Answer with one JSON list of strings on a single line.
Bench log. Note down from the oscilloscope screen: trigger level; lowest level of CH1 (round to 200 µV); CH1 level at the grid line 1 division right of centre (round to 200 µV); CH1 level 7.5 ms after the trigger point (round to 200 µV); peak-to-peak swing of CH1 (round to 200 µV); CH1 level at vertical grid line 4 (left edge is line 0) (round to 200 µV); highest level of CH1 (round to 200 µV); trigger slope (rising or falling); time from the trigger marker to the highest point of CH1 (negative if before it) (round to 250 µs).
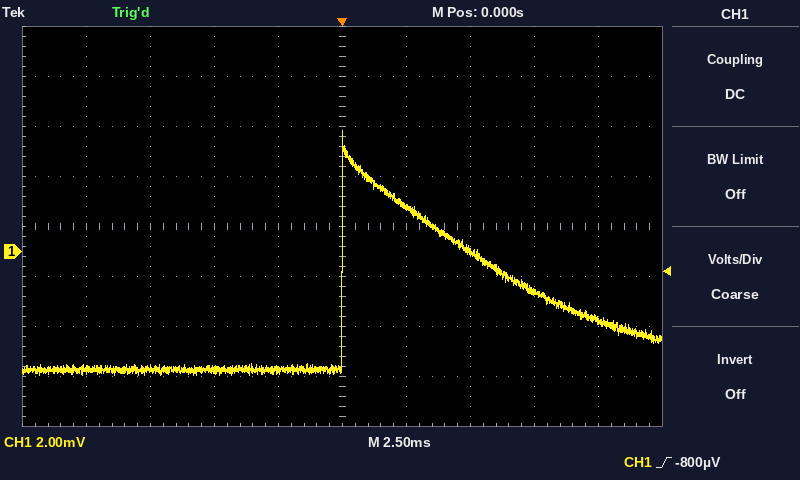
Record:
["-800 µV", "-5.0 mV", "1.8 mV", "-1.6 mV", "9.8 mV", "-4.8 mV", "4.8 mV", "rising", "0.00 ms"]
